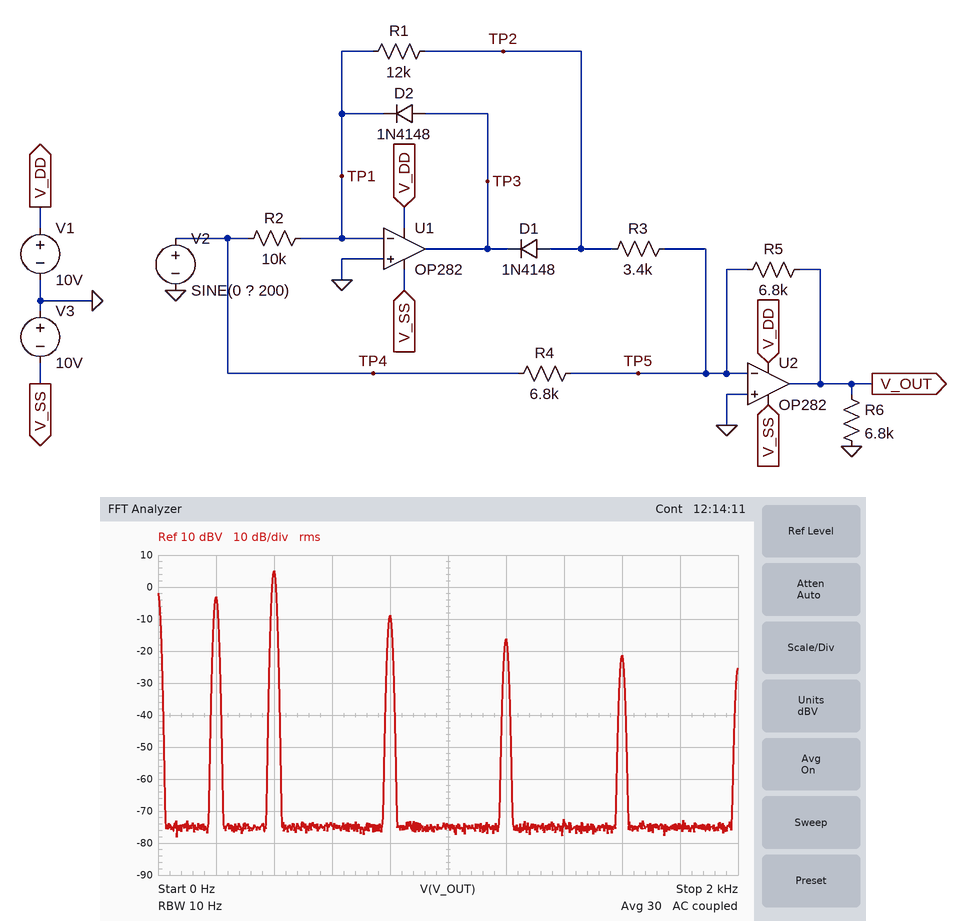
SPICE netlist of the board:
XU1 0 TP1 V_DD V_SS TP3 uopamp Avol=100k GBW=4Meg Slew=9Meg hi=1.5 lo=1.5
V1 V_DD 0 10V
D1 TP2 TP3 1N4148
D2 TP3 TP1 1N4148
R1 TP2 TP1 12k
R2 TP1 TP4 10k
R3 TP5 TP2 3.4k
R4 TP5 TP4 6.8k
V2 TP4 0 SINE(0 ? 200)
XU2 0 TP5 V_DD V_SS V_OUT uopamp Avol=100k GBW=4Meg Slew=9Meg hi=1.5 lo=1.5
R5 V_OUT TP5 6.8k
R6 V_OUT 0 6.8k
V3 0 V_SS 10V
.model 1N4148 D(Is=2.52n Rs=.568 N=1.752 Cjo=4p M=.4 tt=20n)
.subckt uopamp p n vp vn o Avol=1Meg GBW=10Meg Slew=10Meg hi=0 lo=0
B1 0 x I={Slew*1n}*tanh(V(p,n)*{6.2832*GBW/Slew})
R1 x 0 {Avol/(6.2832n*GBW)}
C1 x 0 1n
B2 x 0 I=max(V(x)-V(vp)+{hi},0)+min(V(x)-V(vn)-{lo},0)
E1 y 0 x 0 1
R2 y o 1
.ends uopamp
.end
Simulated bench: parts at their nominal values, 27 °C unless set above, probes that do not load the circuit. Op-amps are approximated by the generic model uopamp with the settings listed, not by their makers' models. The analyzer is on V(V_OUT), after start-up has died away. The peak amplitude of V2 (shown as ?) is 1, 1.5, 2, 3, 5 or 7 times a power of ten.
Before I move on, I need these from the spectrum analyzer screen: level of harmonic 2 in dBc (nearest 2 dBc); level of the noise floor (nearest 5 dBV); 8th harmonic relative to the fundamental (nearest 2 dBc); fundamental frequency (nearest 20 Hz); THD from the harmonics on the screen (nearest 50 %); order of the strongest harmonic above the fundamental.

8 dBc
-75 dBV
-18 dBc
200 Hz
250 %
2
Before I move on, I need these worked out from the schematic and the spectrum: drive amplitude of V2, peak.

5 V
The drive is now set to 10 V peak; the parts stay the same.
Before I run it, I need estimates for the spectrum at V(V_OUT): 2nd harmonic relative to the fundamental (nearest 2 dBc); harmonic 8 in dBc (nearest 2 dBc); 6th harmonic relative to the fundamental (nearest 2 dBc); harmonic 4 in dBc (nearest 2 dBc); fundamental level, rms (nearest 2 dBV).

16 dBc
-10 dBc
2 dBc
12 dBc
-10 dBV
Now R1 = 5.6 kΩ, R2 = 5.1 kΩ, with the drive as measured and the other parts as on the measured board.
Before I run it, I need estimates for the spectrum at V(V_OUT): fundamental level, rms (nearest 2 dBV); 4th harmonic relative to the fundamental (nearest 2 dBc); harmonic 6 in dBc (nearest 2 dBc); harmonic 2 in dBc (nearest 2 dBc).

-10 dBV
0 dBc
-8 dBc
14 dBc
